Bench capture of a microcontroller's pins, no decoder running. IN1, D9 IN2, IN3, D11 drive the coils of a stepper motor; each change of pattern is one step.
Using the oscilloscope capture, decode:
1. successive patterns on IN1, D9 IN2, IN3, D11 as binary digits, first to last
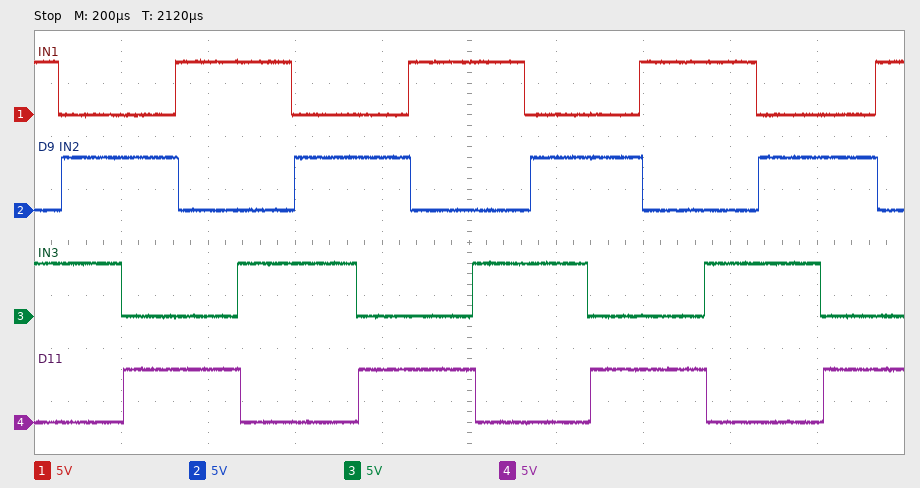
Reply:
1010 0110 0101 1001 1010 0110 0101 1001 1010 0110 0101 1001 1010 0110 0101 1001
